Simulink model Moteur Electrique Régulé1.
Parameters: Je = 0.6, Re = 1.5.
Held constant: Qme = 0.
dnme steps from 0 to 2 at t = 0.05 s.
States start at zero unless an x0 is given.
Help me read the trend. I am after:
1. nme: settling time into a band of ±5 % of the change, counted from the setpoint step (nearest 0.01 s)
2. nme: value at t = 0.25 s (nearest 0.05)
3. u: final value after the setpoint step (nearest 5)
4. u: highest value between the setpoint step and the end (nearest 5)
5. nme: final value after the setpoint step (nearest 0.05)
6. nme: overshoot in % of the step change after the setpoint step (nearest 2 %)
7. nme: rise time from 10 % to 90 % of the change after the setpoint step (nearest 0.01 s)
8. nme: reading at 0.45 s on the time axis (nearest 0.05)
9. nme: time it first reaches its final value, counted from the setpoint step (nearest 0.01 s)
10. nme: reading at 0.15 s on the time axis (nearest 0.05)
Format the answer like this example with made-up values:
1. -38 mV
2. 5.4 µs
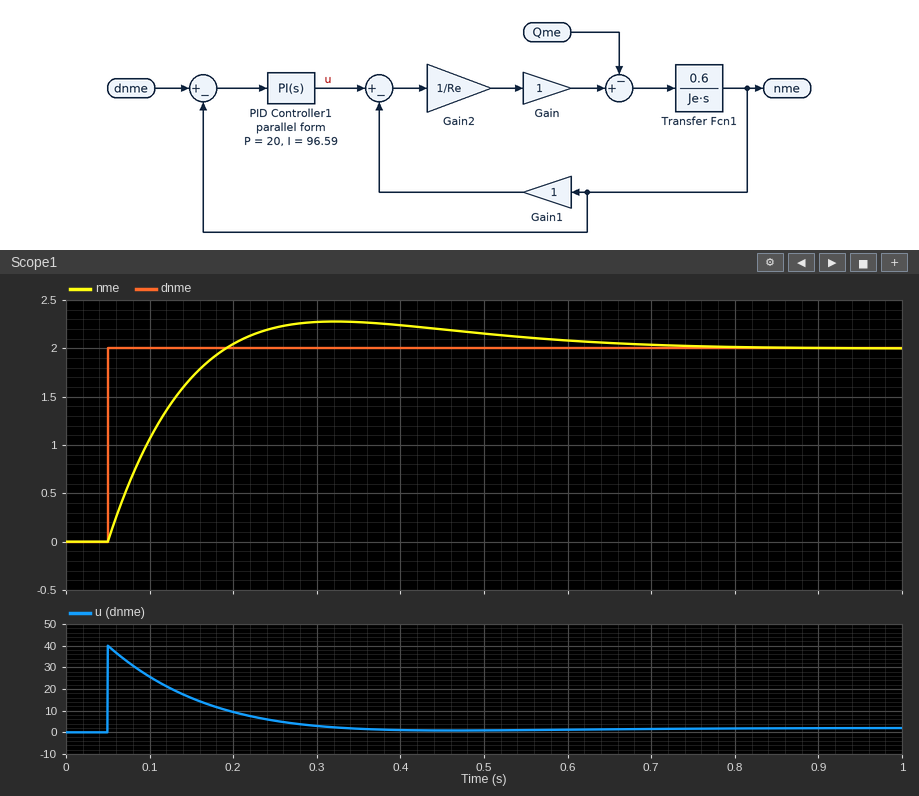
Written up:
1. 0.52 s
2. 2.20
3. 0
4. 40
5. 2.00
6. 14 %
7. 0.10 s
8. 2.20
9. 0.14 s
10. 1.70
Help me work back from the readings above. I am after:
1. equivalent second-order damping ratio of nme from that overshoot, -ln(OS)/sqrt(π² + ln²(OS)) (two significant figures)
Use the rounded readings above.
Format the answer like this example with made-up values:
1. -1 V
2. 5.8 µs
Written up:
1. 0.53
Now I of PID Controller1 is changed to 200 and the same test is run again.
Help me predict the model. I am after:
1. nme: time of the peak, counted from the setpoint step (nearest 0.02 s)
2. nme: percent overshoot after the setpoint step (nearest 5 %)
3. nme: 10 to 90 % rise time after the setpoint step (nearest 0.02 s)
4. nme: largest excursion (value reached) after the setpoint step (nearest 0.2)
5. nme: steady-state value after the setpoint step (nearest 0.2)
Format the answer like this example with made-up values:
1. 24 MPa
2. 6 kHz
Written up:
1. 0.20 s
2. 25 %
3. 0.08 s
4. 2.4
5. 2.0
